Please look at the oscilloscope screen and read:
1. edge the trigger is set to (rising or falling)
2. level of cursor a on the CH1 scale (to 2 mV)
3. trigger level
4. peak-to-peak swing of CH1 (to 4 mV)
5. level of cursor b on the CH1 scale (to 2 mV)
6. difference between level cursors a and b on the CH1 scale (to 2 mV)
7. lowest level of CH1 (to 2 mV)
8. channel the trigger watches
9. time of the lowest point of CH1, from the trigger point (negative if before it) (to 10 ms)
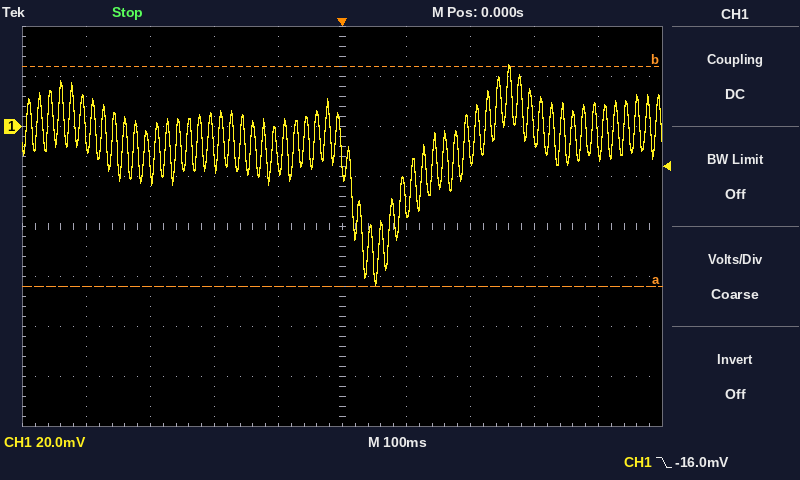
falling
-64 mV
-16.0 mV
88 mV
24 mV
88 mV
-64 mV
CH1
+50 ms
